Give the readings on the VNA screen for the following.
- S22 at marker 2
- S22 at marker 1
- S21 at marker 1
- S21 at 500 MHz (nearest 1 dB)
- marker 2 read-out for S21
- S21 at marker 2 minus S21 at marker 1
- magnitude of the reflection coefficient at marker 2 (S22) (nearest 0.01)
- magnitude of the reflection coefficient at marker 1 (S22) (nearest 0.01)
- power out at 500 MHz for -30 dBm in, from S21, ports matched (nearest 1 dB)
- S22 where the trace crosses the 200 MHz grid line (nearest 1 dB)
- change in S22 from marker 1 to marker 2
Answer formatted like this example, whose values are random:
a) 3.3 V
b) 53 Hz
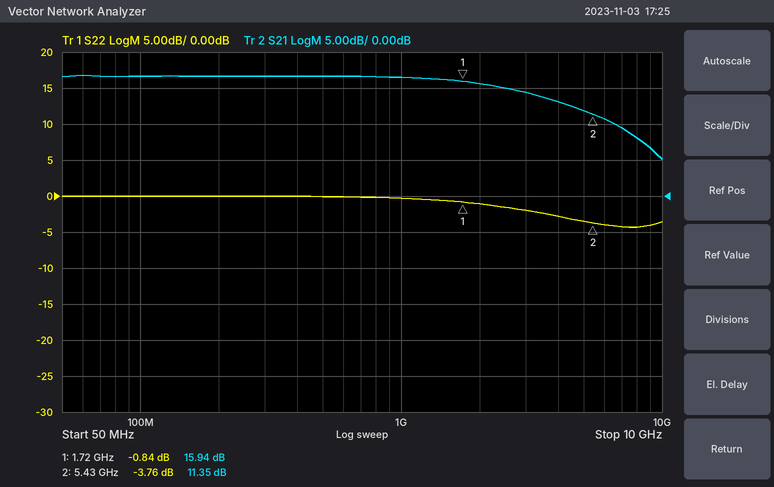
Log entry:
a) -3.76 dB
b) -0.84 dB
c) 15.94 dB
d) 17 dB
e) 11.35 dB
f) -4.59 dB
g) 0.65
h) 0.91
i) -13 dBm
j) 0 dB
k) -2.92 dB
